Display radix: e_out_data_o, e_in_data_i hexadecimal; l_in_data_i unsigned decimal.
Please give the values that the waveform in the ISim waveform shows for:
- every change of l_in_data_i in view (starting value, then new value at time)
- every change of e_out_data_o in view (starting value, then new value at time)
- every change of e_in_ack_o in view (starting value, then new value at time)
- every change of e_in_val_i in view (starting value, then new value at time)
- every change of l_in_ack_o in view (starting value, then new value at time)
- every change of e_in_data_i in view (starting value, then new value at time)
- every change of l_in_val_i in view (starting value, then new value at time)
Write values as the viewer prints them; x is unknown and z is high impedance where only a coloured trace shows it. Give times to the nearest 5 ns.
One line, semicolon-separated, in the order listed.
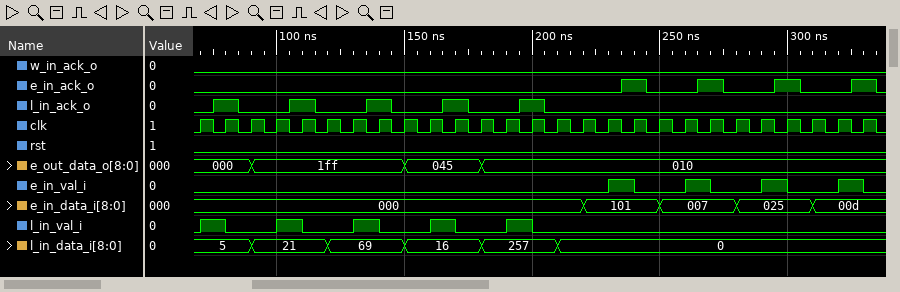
5, 21 at 90 ns, 69 at 120 ns, 16 at 150 ns, 257 at 180 ns, 0 at 210 ns; 000, 1ff at 90 ns, 045 at 150 ns, 010 at 180 ns; 0, 1 at 235 ns, 0 at 245 ns, 1 at 265 ns, 0 at 275 ns, 1 at 295 ns, 0 at 305 ns, 1 at 325 ns, 0 at 335 ns; 0, 1 at 230 ns, 0 at 240 ns, 1 at 260 ns, 0 at 270 ns, 1 at 290 ns, 0 at 300 ns, 1 at 320 ns, 0 at 330 ns; 0, 1 at 75 ns, 0 at 85 ns, 1 at 105 ns, 0 at 115 ns, 1 at 135 ns, 0 at 145 ns, 1 at 165 ns, 0 at 175 ns, 1 at 195 ns, 0 at 205 ns; 000, 101 at 220 ns, 007 at 250 ns, 025 at 280 ns, 00d at 310 ns; 0, 1 at 70 ns, 0 at 80 ns, 1 at 100 ns, 0 at 110 ns, 1 at 130 ns, 0 at 140 ns, 1 at 160 ns, 0 at 170 ns, 1 at 190 ns, 0 at 200 ns
